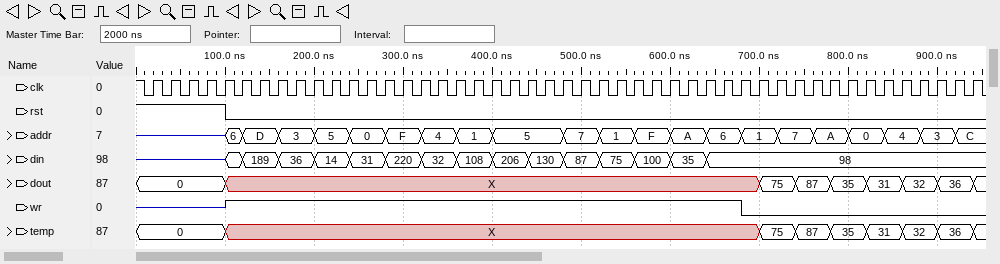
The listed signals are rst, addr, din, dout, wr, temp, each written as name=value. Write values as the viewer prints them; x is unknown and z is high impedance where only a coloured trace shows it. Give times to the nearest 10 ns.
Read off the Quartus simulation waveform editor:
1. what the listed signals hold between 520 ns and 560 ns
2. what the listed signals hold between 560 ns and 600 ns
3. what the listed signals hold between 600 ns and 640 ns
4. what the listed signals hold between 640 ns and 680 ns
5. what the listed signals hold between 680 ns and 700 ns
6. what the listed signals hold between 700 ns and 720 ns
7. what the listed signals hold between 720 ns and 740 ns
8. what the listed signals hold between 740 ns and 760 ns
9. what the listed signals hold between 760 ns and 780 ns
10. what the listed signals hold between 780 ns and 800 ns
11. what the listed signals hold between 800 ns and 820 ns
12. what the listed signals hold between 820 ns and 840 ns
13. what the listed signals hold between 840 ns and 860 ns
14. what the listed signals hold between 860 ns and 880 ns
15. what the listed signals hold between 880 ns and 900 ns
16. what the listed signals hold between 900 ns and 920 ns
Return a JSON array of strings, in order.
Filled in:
["rst=0, addr=1, din=75, dout=X, wr=1, temp=X", "rst=0, addr=F, din=100, dout=X, wr=1, temp=X", "rst=0, addr=A, din=35, dout=X, wr=1, temp=X", "rst=0, addr=6, din=98, dout=X, wr=1, temp=X", "rst=0, addr=1, din=98, dout=X, wr=0, temp=X", "rst=0, addr=1, din=98, dout=75, wr=0, temp=75", "rst=0, addr=7, din=98, dout=75, wr=0, temp=75", "rst=0, addr=7, din=98, dout=87, wr=0, temp=87", "rst=0, addr=A, din=98, dout=87, wr=0, temp=87", "rst=0, addr=A, din=98, dout=35, wr=0, temp=35", "rst=0, addr=0, din=98, dout=35, wr=0, temp=35", "rst=0, addr=0, din=98, dout=31, wr=0, temp=31", "rst=0, addr=4, din=98, dout=31, wr=0, temp=31", "rst=0, addr=4, din=98, dout=32, wr=0, temp=32", "rst=0, addr=3, din=98, dout=32, wr=0, temp=32", "rst=0, addr=3, din=98, dout=36, wr=0, temp=36"]
